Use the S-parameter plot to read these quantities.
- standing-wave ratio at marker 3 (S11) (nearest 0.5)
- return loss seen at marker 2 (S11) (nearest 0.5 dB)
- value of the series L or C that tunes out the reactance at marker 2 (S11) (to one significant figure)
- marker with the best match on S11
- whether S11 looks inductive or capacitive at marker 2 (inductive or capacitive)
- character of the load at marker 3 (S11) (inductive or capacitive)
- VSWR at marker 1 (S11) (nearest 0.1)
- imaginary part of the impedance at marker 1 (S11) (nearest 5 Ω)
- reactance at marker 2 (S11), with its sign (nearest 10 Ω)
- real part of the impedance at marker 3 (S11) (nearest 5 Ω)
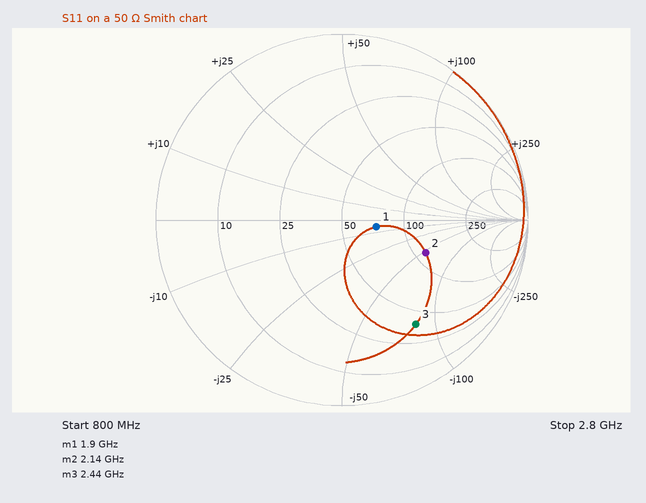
5.5
6.5 dB
4 nH
marker 1
capacitive
capacitive
1.5
-5 Ω
-50 Ω
40 Ω
